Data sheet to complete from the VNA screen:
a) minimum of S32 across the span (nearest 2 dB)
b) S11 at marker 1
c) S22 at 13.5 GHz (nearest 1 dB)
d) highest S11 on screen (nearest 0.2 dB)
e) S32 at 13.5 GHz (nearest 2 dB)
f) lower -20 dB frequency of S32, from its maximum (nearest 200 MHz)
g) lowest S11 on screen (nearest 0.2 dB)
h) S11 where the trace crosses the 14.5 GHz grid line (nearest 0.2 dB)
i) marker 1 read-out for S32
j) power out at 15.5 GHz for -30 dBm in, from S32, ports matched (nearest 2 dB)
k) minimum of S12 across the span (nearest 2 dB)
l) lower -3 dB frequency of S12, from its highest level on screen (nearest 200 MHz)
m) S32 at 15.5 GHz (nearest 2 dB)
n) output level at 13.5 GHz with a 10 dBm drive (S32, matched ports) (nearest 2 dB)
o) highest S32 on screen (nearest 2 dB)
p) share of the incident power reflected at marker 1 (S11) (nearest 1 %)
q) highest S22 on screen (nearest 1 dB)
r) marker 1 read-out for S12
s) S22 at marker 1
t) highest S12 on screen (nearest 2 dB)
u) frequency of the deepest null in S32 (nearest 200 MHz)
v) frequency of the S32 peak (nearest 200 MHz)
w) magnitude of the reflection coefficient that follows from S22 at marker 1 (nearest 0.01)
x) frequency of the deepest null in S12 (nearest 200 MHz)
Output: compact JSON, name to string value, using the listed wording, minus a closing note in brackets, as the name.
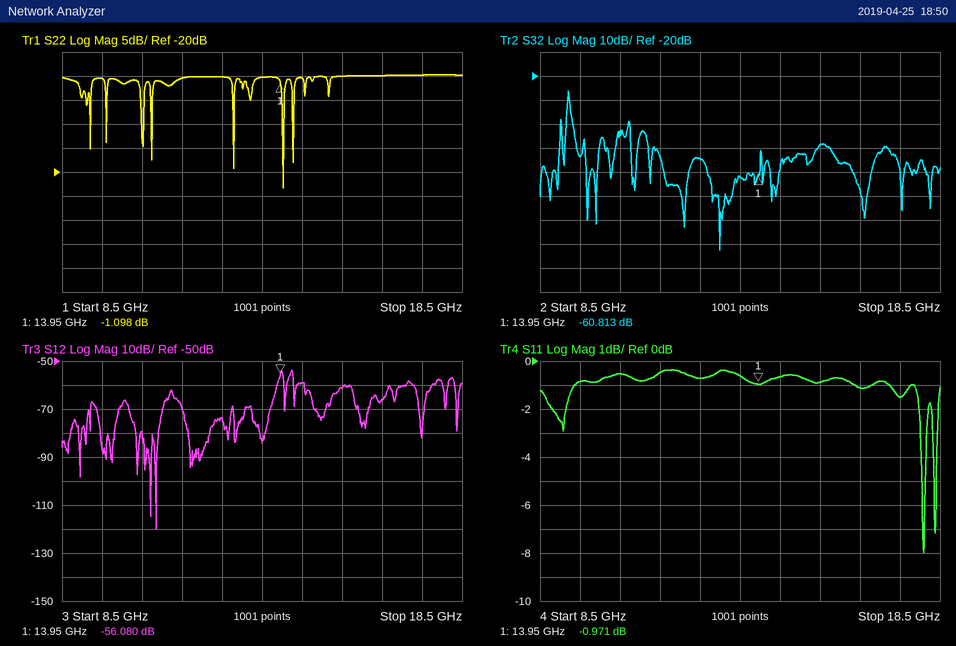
{"minimum of S32 across the span": "-92 dB", "S11 at marker 1": "-0.971 dB", "S22 at 13.5 GHz": "0 dB", "highest S11 on screen": "-0.4 dB", "S32 at 13.5 GHz": "-62 dB", "lower -20 dB frequency of S32, from its maximum": "9.2 GHz", "lowest S11 on screen": "-8.0 dB", "S11 where the trace crosses the 14.5 GHz grid line": "-0.6 dB", "marker 1 read-out for S32": "-60.813 dB", "power out at 15.5 GHz for -30 dBm in, from S32, ports matched": "-78 dBm", "minimum of S12 across the span": "-120 dB", "lower -3 dB frequency of S12, from its highest level on screen": "14.2 GHz", "S32 at 15.5 GHz": "-48 dB", "output level at 13.5 GHz with a 10 dBm drive (S32, matched ports)": "-52 dBm", "highest S32 on screen": "-26 dB", "share of the incident power reflected at marker 1 (S11)": "80 %", "highest S22 on screen": "0 dB", "marker 1 read-out for S12": "-56.080 dB", "S22 at marker 1": "-1.098 dB", "highest S12 on screen": "-54 dB", "frequency of the deepest null in S32": "13.0 GHz", "frequency of the S32 peak": "9.2 GHz", "magnitude of the reflection coefficient that follows from S22 at marker 1": "0.88", "frequency of the deepest null in S12": "10.8 GHz"}
